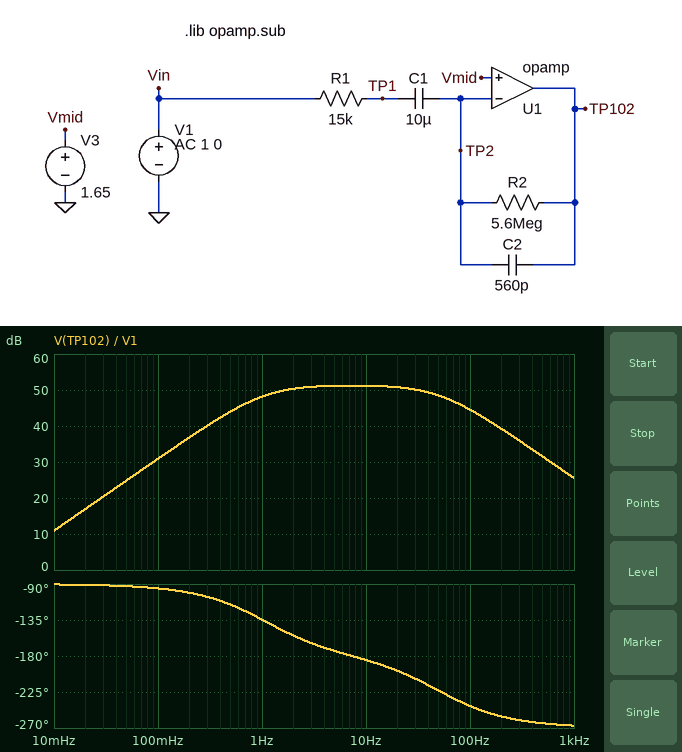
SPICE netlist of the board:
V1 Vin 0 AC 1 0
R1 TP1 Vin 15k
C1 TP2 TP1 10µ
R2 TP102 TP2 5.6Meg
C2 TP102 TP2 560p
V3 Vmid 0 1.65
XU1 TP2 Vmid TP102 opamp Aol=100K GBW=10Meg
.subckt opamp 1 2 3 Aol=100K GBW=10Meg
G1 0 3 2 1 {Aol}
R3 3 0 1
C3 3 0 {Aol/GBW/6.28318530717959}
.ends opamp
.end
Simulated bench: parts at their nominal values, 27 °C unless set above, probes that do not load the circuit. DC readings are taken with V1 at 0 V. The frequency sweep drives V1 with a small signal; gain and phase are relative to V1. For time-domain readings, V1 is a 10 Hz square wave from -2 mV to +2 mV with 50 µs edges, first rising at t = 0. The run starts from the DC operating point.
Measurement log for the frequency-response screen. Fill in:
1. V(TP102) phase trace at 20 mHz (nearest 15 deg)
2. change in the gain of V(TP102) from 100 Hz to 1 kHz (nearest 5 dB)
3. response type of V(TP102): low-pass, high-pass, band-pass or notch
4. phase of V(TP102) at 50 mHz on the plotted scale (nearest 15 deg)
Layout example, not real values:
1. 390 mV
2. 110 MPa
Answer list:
1. -90 deg
2. -20 dB
3. band-pass
4. -90 deg
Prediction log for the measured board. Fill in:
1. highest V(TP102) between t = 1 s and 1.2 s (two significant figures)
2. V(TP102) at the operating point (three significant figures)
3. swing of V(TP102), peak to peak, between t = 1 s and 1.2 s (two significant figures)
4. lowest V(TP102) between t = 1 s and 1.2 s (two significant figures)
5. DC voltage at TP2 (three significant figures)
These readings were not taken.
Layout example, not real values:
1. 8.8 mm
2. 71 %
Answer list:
1. 2.4 V
2. 1.65 V
3. 1.6 V
4. 860 mV
5. 1.65 V
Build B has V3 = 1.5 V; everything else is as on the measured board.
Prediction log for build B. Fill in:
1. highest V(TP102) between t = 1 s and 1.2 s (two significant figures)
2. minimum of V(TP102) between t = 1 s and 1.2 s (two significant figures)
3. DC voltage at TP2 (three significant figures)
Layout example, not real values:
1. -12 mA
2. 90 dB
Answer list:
1. 2.3 V
2. 710 mV
3. 1.50 V
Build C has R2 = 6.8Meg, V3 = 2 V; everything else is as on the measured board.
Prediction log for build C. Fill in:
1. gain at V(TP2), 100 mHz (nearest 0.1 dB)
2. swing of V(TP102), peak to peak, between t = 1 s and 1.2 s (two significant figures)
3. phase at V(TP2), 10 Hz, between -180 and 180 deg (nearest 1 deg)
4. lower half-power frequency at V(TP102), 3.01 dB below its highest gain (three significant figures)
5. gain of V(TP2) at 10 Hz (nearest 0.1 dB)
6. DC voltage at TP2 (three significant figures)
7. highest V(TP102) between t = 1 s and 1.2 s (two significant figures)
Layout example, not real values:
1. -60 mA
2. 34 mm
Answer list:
1. -67.4 dB
2. 1.9 V
3. -2 deg
4. 1.01 Hz
5. -47.2 dB
6. 2.00 V
7. 2.9 V
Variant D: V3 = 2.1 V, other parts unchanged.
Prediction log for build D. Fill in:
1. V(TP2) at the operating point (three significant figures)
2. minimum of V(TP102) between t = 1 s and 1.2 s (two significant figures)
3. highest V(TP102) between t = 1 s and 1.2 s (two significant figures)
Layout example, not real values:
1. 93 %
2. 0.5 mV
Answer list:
1. 2.10 V
2. 1.3 V
3. 2.9 V
